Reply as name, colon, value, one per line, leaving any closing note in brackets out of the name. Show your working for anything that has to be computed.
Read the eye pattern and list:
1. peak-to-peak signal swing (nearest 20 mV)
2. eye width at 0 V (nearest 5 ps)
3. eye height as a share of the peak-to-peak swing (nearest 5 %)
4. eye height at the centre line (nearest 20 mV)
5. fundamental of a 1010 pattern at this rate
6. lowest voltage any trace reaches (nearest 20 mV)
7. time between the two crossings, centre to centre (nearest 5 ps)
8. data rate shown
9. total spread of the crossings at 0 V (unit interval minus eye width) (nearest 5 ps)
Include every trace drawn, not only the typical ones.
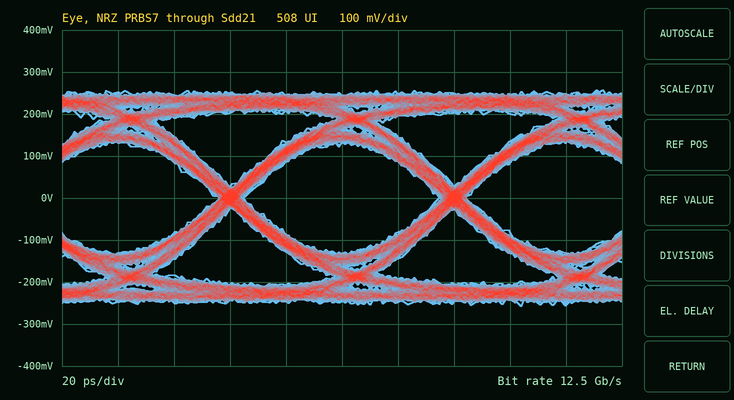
peak-to-peak signal swing: 520 mV
eye width at 0 V: 70 ps
eye height as a share of the peak-to-peak swing: 260 mV / 520 mV ≈ 50 %
eye height at the centre line: 260 mV
fundamental of a 1010 pattern at this rate: 6.25 GHz
lowest voltage any trace reaches: -260 mV
time between the two crossings, centre to centre: 80 ps
data rate shown: 12.5 Gb/s
total spread of the crossings at 0 V (unit interval minus eye width): 10 ps
